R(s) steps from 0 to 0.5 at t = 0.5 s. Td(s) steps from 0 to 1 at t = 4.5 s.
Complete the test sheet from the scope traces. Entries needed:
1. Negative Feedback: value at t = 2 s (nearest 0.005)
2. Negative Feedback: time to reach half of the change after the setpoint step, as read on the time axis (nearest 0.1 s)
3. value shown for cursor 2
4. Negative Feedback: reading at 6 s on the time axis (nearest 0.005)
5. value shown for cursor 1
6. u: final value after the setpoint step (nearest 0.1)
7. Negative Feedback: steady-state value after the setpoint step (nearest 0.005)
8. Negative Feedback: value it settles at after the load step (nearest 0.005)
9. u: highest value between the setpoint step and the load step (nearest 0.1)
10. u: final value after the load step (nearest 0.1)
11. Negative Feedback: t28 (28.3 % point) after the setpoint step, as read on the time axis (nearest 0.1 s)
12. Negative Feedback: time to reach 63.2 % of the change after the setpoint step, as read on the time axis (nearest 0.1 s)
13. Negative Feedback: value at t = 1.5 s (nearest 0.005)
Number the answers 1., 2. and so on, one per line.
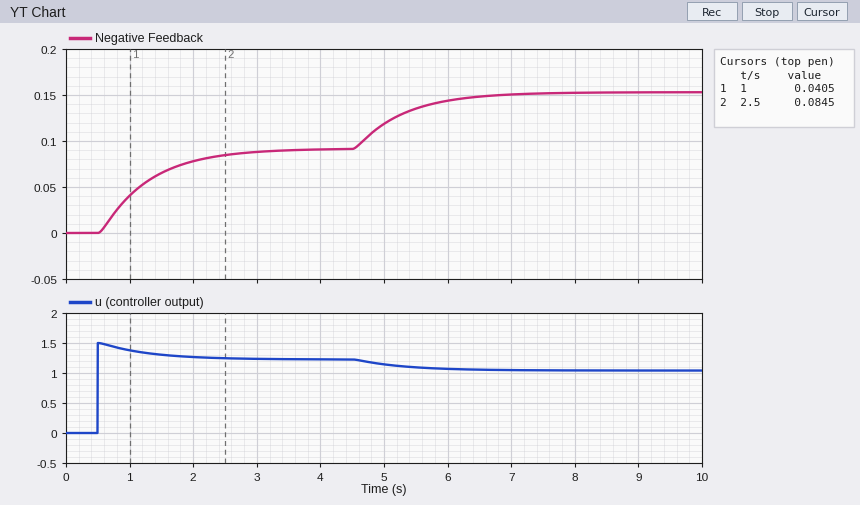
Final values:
1. 0.080
2. 1.1 s
3. 0.0845
4. 0.145
5. 0.0405
6. 1.2
7. 0.090
8. 0.155
9. 1.5
10. 1.0
11. 0.8 s
12. 1.3 s
13. 0.065
